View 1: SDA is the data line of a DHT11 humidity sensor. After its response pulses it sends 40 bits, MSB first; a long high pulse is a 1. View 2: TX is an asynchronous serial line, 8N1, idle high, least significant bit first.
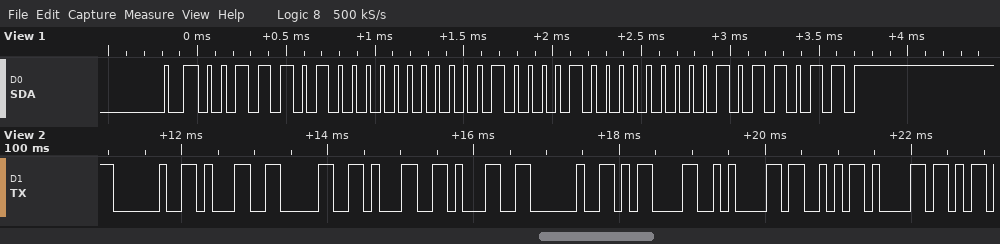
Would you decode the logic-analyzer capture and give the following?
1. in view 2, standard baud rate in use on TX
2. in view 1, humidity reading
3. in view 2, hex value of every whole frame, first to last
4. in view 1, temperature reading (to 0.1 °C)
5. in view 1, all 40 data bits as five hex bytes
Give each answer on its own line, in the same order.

9600 baud
58 %
0x20 0x31 0x30 0x31 0x31 0x20 0x0D 0x0A 0x53 0x61
33.0 °C
3A 00 21 00 5B
